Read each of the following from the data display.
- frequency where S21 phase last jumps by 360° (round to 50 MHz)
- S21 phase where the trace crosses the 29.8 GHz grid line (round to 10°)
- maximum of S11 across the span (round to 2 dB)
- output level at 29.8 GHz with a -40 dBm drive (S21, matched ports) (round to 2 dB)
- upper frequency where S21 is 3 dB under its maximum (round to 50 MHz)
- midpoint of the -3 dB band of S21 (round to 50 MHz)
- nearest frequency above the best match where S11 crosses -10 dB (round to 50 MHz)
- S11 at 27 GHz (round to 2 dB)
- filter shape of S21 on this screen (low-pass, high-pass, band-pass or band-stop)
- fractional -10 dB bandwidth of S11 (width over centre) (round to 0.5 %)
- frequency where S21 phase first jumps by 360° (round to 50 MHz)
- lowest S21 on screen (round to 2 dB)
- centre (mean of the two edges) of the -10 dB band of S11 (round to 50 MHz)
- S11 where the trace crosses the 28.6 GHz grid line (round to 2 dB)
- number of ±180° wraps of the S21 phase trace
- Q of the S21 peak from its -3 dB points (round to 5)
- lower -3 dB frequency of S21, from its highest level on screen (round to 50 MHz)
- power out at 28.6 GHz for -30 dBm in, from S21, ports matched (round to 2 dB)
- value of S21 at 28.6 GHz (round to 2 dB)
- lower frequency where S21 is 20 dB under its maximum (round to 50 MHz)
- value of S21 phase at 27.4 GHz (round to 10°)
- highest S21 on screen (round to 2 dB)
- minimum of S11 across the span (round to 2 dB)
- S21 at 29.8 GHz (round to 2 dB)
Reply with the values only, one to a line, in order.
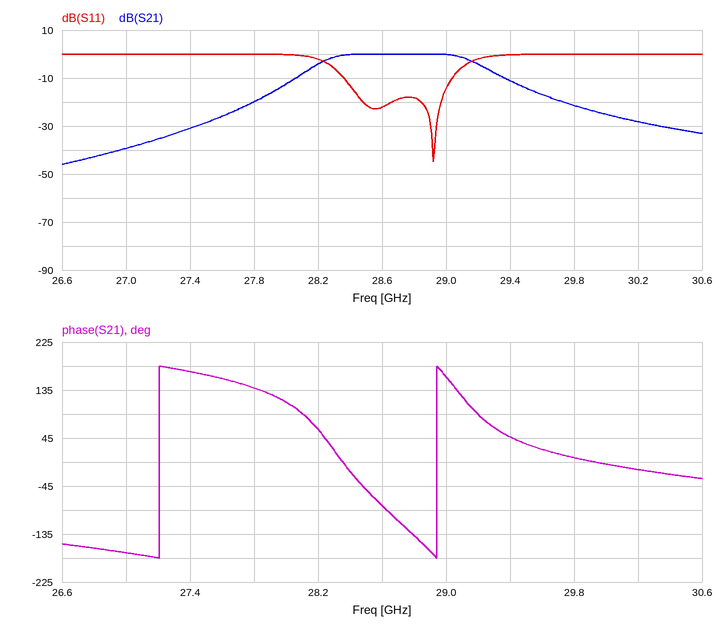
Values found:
28.95 GHz
10°
0 dB
-62 dBm
29.15 GHz
28.70 GHz
29.05 GHz
0 dB
band-pass
2.5 %
27.20 GHz
-46 dB
28.70 GHz
-22 dB
2
30
28.25 GHz
-30 dBm
0 dB
27.80 GHz
170°
0 dB
-44 dB
-22 dB
